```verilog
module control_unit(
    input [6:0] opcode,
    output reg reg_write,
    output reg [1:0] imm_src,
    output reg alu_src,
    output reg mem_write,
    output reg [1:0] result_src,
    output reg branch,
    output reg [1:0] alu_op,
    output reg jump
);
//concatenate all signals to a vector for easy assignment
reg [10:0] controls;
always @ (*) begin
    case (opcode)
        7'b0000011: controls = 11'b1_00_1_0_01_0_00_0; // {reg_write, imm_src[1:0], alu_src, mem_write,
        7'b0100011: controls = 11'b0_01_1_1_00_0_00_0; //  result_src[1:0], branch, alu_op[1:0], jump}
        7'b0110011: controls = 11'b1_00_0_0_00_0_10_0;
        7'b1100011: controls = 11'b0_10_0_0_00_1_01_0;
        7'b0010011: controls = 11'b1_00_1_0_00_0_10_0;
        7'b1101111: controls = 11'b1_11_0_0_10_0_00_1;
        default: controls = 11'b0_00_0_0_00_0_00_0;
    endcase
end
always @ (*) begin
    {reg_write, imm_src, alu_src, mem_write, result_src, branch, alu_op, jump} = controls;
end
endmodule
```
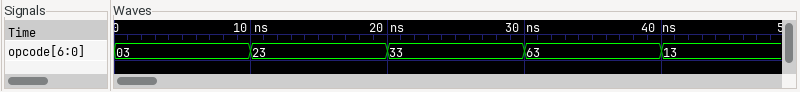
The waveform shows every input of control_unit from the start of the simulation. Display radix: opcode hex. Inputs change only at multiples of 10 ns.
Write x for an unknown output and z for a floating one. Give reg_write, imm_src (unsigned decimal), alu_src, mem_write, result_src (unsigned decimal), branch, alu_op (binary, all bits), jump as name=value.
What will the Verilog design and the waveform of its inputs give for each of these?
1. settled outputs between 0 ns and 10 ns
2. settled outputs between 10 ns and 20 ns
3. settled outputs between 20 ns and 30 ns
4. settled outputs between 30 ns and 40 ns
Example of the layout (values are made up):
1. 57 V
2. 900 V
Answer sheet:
1. reg_write=1, imm_src=0, alu_src=1, mem_write=0, result_src=1, branch=0, alu_op=00, jump=0
2. reg_write=0, imm_src=1, alu_src=1, mem_write=1, result_src=0, branch=0, alu_op=00, jump=0
3. reg_write=1, imm_src=0, alu_src=0, mem_write=0, result_src=0, branch=0, alu_op=10, jump=0
4. reg_write=0, imm_src=2, alu_src=0, mem_write=0, result_src=0, branch=1, alu_op=01, jump=0
